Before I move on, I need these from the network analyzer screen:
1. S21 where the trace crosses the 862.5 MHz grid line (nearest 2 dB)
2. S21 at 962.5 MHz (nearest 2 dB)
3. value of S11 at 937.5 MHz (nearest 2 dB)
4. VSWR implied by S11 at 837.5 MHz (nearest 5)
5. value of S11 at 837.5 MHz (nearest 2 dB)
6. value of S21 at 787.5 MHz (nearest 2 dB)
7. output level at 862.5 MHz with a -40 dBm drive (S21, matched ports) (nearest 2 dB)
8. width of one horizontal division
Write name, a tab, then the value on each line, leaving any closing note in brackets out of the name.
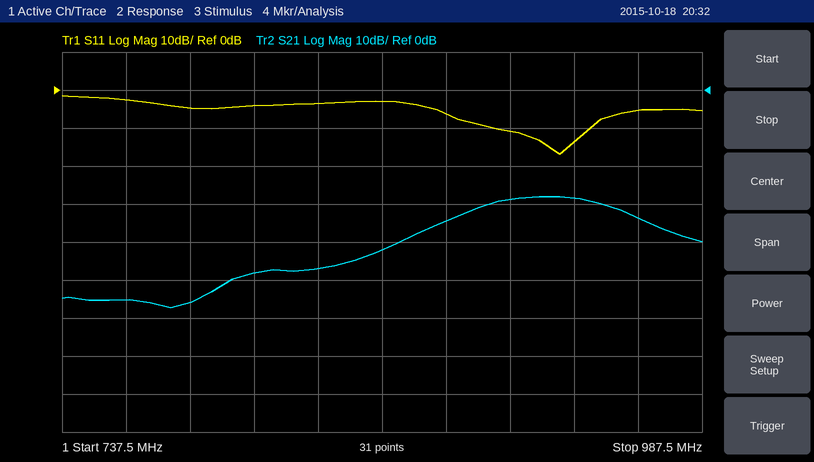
S21 where the trace crosses the 862.5 MHz grid line	-42 dB
S21 at 962.5 MHz	-34 dB
value of S11 at 937.5 MHz	-14 dB
VSWR implied by S11 at 837.5 MHz	5
value of S11 at 837.5 MHz	-4 dB
value of S21 at 787.5 MHz	-56 dB
output level at 862.5 MHz with a -40 dBm drive (S21, matched ports)	-82 dBm
width of one horizontal division	25 MHz
